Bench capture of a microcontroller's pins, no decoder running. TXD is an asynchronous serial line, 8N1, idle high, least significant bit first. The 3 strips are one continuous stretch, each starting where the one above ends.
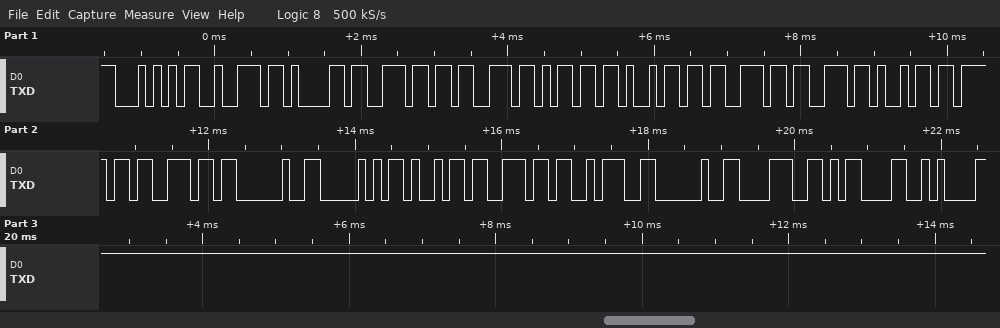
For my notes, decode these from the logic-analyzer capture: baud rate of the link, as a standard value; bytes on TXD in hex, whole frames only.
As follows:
9600 baud
0x54 0x72 0x61 0x6E 0x73 0x6D 0x69 0x73 0x73 0x69 0x6F 0x6E 0x20 0x50 0x69 0x6E 0x3A 0x20 0x38 0x0D 0x0A
